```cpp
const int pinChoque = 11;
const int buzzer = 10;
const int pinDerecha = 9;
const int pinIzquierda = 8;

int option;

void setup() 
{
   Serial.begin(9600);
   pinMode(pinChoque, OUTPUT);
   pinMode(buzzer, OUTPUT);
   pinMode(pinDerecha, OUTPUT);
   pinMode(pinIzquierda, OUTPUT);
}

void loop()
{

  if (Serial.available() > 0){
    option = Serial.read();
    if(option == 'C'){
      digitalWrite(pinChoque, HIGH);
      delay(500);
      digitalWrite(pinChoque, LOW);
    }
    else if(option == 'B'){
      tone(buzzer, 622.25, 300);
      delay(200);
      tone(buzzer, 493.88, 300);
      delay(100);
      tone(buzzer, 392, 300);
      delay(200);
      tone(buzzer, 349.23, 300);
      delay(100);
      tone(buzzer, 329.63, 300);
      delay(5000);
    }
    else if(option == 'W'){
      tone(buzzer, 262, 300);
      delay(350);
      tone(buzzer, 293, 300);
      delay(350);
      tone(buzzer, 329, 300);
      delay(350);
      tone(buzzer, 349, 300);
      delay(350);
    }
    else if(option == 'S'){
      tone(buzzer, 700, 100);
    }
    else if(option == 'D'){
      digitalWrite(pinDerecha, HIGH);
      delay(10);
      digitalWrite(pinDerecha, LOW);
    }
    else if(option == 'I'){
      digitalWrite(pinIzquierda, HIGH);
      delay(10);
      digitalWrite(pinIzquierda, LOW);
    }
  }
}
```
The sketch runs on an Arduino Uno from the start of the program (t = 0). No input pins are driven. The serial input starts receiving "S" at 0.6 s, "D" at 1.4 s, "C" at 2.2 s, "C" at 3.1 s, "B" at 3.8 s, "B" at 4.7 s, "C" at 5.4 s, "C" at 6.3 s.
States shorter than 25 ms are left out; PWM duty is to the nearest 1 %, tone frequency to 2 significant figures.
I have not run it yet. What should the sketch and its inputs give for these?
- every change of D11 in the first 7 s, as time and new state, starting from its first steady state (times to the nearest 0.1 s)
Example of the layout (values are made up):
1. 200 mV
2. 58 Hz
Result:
1. 0 s low; 2.2 s high; 2.7 s low; 3.1 s high; 3.6 s low
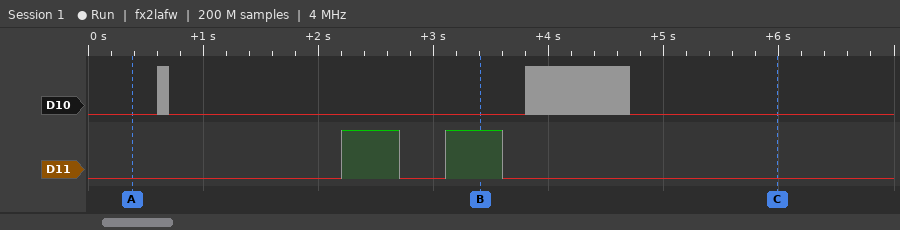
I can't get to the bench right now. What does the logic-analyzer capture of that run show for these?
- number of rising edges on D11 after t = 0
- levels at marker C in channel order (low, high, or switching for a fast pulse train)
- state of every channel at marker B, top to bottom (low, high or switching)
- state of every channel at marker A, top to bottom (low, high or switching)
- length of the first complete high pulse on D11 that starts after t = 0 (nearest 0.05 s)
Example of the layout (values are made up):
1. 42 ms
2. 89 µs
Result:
1. 2
2. D10 low, D11 low
3. D10 low, D11 high
4. D10 low, D11 low
5. 0.50 s
